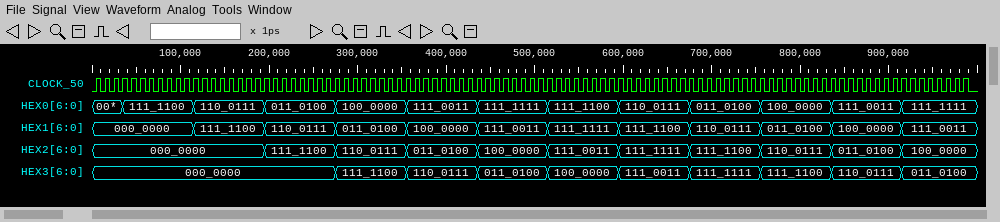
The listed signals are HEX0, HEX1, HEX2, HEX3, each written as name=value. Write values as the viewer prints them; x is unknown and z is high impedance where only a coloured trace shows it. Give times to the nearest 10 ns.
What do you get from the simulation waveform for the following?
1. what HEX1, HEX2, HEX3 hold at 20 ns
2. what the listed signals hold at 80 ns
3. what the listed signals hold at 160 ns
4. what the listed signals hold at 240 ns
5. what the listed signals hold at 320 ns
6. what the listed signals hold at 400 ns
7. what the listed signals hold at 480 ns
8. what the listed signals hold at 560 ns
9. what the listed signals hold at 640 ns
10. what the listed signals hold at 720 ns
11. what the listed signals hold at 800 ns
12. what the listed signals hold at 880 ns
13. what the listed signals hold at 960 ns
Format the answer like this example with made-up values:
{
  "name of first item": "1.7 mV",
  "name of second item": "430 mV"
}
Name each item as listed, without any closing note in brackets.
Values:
{
  "what HEX1, HEX2, HEX3 hold at 20 ns": "HEX1=000_0000, HEX2=000_0000, HEX3=000_0000",
  "what the listed signals hold at 80 ns": "HEX0=111_1100, HEX1=000_0000, HEX2=000_0000, HEX3=000_0000",
  "what the listed signals hold at 160 ns": "HEX0=110_0111, HEX1=111_1100, HEX2=000_0000, HEX3=000_0000",
  "what the listed signals hold at 240 ns": "HEX0=011_0100, HEX1=110_0111, HEX2=111_1100, HEX3=000_0000",
  "what the listed signals hold at 320 ns": "HEX0=100_0000, HEX1=011_0100, HEX2=110_0111, HEX3=111_1100",
  "what the listed signals hold at 400 ns": "HEX0=111_0011, HEX1=100_0000, HEX2=011_0100, HEX3=110_0111",
  "what the listed signals hold at 480 ns": "HEX0=111_1111, HEX1=111_0011, HEX2=100_0000, HEX3=011_0100",
  "what the listed signals hold at 560 ns": "HEX0=111_1100, HEX1=111_1111, HEX2=111_0011, HEX3=100_0000",
  "what the listed signals hold at 640 ns": "HEX0=110_0111, HEX1=111_1100, HEX2=111_1111, HEX3=111_0011",
  "what the listed signals hold at 720 ns": "HEX0=011_0100, HEX1=110_0111, HEX2=111_1100, HEX3=111_1111",
  "what the listed signals hold at 800 ns": "HEX0=100_0000, HEX1=011_0100, HEX2=110_0111, HEX3=111_1100",
  "what the listed signals hold at 880 ns": "HEX0=111_0011, HEX1=100_0000, HEX2=011_0100, HEX3=110_0111",
  "what the listed signals hold at 960 ns": "HEX0=111_1111, HEX1=111_0011, HEX2=100_0000, HEX3=011_0100"
}
